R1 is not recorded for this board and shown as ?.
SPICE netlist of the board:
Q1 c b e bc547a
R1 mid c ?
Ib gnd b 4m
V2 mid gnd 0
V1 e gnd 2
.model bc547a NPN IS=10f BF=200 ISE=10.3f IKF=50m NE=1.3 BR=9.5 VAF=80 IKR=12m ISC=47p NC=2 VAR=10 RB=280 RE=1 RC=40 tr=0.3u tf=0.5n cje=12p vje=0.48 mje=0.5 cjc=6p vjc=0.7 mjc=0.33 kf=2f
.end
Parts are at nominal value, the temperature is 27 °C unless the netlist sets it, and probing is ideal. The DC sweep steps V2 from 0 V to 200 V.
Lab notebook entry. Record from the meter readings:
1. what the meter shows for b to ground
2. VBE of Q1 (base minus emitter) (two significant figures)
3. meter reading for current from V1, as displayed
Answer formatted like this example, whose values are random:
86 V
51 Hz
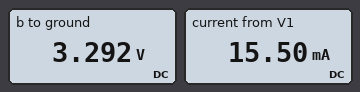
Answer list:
3.292 V
1.3 V
15.50 mA
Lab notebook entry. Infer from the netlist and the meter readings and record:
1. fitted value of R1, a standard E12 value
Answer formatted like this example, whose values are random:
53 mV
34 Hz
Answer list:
33 Ω
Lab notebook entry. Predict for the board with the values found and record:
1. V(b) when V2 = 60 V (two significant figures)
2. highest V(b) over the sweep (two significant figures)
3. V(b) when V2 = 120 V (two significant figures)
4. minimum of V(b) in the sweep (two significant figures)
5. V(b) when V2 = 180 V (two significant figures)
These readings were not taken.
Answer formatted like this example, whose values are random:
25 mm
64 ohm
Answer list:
4.2 V
4.4 V
4.3 V
3.3 V
4.4 V
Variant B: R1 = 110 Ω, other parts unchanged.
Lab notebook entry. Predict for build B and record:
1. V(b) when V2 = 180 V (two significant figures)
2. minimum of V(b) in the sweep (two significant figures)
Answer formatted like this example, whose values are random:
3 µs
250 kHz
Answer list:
4.3 V
3.8 V
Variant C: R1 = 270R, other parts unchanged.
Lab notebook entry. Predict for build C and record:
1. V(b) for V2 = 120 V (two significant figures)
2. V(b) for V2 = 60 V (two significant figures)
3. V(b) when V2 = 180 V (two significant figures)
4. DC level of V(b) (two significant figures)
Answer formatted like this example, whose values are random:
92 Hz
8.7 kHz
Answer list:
4.2 V
4.1 V
4.3 V
3.9 V
